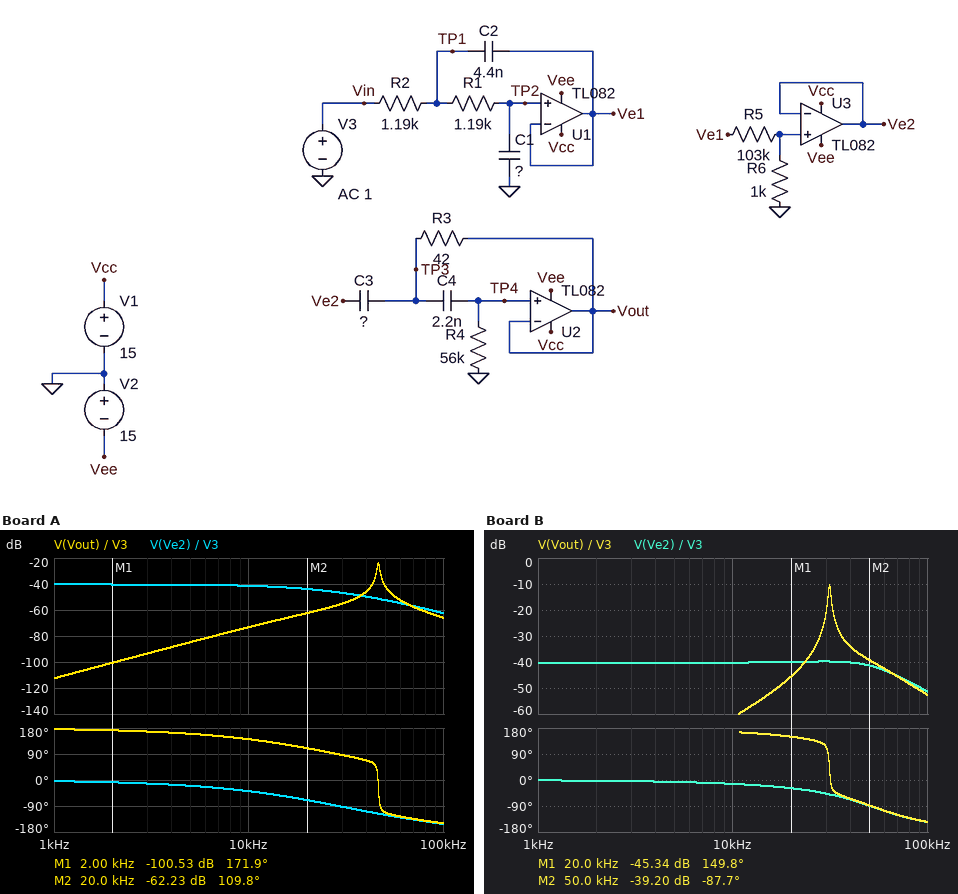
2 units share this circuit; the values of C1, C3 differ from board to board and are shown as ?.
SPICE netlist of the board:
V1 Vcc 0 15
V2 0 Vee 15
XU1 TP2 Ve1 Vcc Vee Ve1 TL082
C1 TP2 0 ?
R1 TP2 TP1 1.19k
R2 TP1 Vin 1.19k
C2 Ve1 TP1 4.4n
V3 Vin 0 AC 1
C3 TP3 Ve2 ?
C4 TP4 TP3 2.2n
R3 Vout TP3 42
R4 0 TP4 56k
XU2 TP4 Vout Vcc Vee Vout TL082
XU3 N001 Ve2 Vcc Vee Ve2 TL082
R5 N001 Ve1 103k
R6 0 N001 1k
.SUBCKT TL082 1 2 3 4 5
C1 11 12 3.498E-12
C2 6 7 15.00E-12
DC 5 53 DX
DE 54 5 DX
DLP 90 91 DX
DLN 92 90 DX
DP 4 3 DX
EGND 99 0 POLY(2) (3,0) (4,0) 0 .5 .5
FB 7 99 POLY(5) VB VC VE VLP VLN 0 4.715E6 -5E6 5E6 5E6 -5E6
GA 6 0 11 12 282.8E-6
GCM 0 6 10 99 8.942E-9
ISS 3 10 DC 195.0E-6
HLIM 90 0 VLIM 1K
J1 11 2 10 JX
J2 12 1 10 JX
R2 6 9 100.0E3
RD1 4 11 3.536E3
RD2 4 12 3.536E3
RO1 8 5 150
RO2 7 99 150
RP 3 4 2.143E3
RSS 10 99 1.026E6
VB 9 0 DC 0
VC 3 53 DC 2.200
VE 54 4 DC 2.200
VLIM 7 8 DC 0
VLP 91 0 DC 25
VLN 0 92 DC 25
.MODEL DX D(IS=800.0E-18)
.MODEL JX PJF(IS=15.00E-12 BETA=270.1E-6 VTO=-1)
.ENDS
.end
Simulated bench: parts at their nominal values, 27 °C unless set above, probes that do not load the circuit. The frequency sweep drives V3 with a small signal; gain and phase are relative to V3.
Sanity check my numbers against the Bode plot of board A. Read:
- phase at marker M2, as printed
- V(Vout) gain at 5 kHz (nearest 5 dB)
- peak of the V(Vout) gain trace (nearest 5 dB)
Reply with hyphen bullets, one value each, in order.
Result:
- 109.8 deg
- -85 dB
- -25 dB
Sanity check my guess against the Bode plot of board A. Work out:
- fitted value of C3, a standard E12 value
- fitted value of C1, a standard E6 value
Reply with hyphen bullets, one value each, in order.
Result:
- 1.2 nF
- 4.7 nF
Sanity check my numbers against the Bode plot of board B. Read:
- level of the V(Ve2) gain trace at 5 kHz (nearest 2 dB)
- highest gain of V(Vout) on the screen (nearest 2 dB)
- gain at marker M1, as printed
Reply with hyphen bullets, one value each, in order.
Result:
- -40 dB
- -10 dB
- -45.34 dB
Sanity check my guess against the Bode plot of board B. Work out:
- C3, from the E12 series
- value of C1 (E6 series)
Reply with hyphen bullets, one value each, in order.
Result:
- 3.9 nF
- 1.5 nF
